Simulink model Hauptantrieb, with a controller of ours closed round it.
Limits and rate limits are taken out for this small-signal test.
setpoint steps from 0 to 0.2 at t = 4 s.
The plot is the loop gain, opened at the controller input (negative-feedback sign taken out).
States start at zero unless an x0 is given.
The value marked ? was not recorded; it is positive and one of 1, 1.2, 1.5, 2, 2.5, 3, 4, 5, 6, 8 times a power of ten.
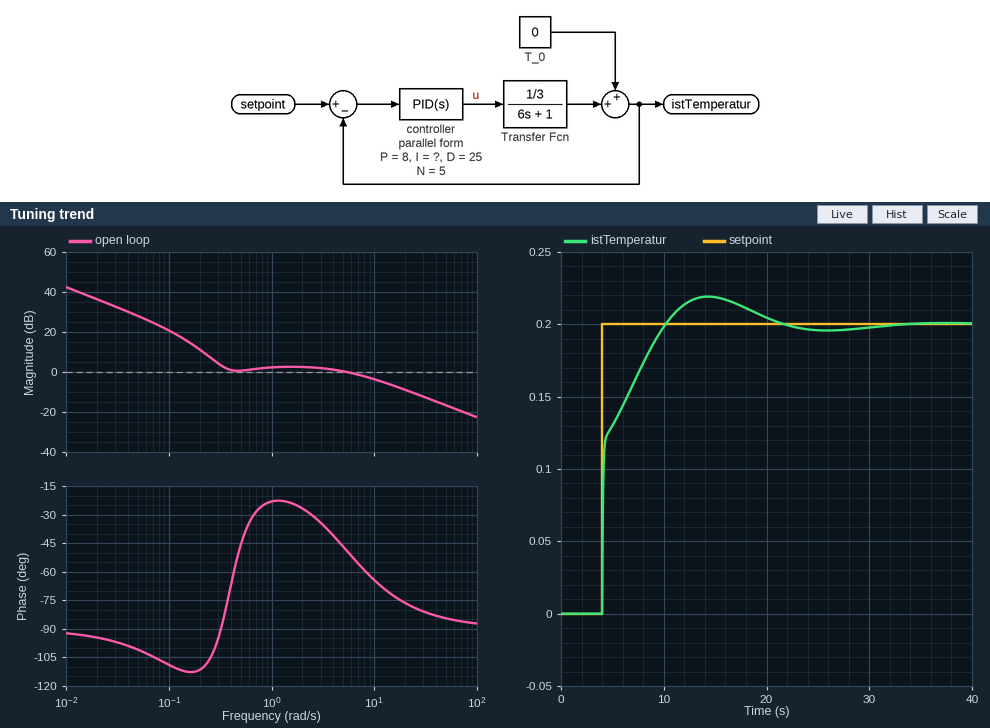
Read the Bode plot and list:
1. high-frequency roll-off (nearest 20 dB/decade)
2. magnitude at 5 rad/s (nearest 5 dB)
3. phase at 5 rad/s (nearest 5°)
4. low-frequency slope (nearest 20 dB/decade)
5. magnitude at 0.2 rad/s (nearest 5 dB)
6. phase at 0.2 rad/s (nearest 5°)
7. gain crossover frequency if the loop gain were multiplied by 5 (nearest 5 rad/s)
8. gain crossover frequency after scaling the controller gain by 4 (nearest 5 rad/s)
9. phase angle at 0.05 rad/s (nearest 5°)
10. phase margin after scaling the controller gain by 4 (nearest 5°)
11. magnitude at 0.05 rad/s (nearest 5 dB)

-20 dB/decade
0 dB
-45°
-20 dB/decade
10 dB
-110°
35 rad/s
30 rad/s
-100°
100°
30 dB
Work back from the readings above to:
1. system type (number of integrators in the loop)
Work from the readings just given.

1
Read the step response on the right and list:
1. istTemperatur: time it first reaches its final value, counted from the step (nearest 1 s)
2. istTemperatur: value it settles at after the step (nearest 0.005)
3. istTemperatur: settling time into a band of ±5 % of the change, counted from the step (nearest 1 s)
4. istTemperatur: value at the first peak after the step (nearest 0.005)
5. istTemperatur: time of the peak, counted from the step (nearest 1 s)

6 s
0.200
14 s
0.220
10 s
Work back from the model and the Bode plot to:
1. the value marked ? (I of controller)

4
